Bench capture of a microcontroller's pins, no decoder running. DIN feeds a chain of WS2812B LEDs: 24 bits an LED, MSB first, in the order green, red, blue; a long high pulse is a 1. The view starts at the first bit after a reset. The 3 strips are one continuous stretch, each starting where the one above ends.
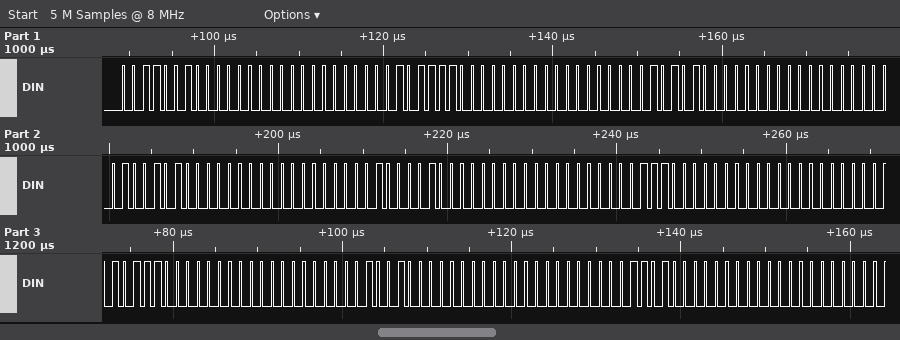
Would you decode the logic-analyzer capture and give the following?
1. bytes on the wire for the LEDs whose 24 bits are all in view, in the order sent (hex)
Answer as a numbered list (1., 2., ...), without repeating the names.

1. 32 00 00 2F 00 00 2A 00 00 25 00 00 21 00 00 1C 00 00 17 00 00 12 00 00 0D 00 00
